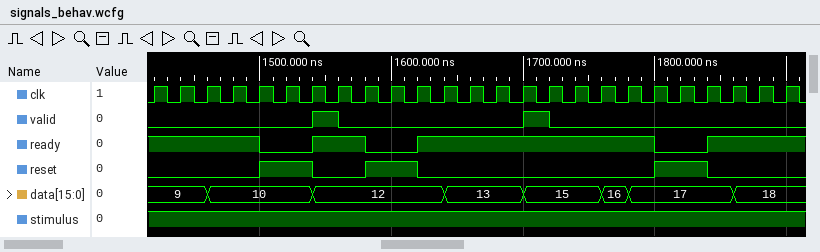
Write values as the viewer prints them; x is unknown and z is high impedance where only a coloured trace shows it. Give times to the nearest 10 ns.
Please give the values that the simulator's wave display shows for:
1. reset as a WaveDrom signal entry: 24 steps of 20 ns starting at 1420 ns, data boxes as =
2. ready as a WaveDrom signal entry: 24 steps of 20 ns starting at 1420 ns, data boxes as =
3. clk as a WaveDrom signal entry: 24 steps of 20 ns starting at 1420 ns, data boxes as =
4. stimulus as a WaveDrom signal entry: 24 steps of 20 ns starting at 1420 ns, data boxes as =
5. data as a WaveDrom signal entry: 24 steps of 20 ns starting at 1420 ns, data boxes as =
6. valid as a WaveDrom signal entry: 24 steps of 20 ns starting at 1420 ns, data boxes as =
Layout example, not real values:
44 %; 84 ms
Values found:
{name: 'reset', wave: '0...1.0.1.0........1.0..'}; {name: 'ready', wave: '1...0.1.0.1........0.1..'}; {name: 'clk', wave: 'p.......................'}; {name: 'stimulus', wave: '1.......................'}; {name: 'data', wave: '=.=...=....=..=..==...=.', data: '9 10 12 13 15 16 17 18'}; {name: 'valid', wave: '0.....10......10........'}
